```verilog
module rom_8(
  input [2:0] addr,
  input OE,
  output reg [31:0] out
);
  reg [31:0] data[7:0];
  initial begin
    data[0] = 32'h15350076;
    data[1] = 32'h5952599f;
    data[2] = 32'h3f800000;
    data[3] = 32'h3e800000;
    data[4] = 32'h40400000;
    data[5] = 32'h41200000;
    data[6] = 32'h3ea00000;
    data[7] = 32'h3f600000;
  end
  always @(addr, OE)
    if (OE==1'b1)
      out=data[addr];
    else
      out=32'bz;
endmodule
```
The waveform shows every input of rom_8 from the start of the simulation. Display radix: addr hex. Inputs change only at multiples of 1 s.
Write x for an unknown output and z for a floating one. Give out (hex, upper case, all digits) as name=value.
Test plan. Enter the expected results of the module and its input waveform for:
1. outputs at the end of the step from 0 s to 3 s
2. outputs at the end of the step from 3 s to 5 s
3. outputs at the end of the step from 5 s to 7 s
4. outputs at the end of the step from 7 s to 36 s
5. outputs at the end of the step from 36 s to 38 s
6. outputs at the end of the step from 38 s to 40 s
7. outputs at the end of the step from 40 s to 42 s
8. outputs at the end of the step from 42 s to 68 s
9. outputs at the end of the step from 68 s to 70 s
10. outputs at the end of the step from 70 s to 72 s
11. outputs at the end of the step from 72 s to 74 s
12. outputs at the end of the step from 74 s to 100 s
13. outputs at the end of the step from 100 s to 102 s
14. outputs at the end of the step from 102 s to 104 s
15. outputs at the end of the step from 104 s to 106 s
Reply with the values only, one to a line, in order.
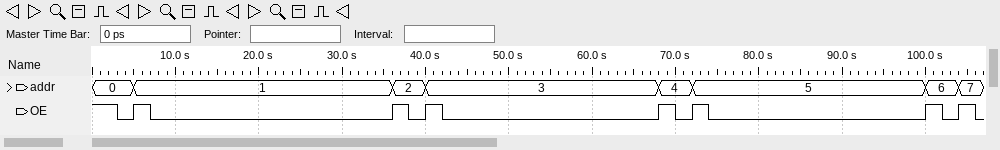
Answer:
out=15350076
out=z
out=5952599F
out=z
out=3F800000
out=z
out=3E800000
out=z
out=40400000
out=z
out=41200000
out=z
out=3EA00000
out=z
out=3F600000
